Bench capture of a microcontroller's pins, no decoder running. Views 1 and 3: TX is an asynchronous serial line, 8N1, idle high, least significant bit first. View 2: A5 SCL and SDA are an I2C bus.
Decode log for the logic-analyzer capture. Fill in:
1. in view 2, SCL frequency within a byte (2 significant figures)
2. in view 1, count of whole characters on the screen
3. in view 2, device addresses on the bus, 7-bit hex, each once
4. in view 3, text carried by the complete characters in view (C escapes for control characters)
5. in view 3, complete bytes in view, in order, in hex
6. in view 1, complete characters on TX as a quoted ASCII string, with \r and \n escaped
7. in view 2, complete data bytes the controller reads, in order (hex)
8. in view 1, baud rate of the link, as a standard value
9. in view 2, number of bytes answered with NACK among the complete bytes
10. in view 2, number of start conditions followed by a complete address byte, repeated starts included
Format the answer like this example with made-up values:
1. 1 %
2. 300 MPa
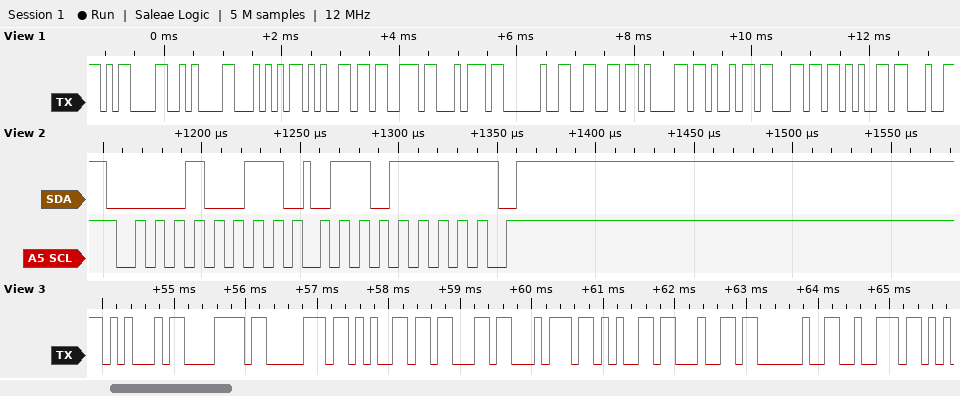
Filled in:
1. 100 kHz
2. 12
3. 0x09
4. "Expected r"
5. 45 78 70 65 63 74 65 64 20 72
6. "\r\nTest faile"
7. 6F
8. 9600 baud
9. 1
10. 1
